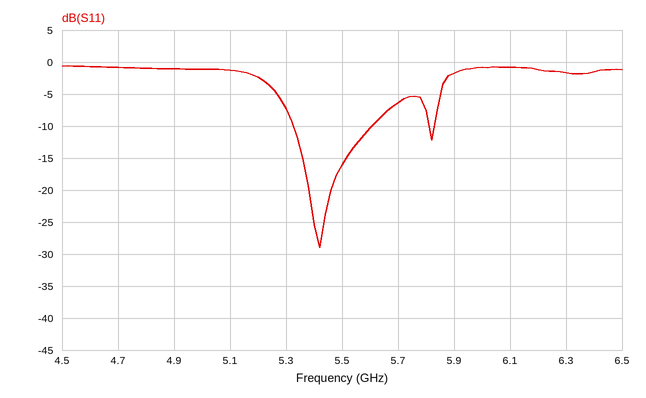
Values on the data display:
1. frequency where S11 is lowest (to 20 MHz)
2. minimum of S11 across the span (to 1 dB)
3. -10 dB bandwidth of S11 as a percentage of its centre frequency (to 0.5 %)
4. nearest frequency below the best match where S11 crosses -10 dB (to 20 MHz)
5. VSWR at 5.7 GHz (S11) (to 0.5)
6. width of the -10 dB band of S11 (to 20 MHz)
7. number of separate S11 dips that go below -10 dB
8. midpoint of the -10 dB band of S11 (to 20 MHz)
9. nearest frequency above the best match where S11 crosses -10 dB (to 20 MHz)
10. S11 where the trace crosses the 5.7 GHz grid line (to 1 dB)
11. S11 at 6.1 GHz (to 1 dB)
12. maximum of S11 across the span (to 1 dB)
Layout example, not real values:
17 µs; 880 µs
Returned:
5.42 GHz; -29 dB; 5.0 %; 5.32 GHz; 3.0; 280 MHz; 2; 5.46 GHz; 5.60 GHz; -6 dB; -1 dB; -1 dB
